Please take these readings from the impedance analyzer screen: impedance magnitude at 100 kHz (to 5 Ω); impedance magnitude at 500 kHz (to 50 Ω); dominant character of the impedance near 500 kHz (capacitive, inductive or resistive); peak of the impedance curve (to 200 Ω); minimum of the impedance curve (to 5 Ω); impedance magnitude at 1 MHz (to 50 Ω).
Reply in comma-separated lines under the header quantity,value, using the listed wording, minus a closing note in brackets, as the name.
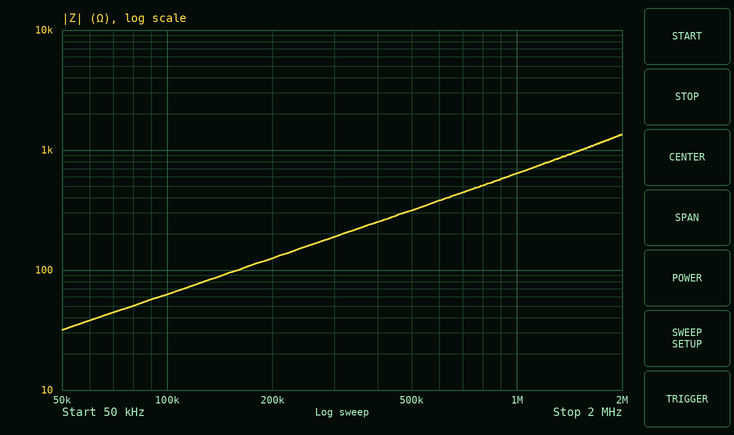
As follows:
quantity,value
impedance magnitude at 100 kHz,65 Ω
impedance magnitude at 500 kHz,300 Ω
dominant character of the impedance near 500 kHz,inductive
peak of the impedance curve,1.4 kΩ
minimum of the impedance curve,30 Ω
impedance magnitude at 1 MHz,650 Ω
